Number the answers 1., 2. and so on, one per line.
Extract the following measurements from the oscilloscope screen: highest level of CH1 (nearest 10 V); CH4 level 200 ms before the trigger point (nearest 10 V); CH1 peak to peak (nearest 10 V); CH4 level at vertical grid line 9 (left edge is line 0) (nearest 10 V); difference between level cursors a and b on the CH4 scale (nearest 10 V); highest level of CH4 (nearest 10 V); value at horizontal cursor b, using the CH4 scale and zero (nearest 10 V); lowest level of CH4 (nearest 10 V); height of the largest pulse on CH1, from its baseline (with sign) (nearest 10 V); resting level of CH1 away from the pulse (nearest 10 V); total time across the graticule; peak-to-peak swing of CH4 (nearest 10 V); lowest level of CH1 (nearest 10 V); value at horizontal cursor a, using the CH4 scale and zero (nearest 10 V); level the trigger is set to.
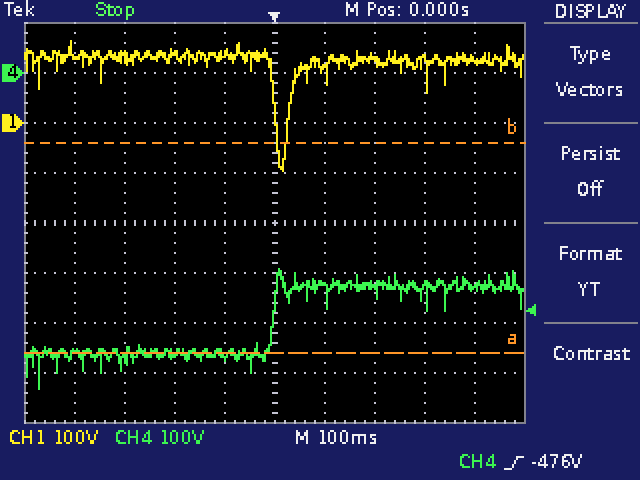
1. 160 V
2. -560 V
3. 260 V
4. -430 V
5. 420 V
6. -390 V
7. -140 V
8. -630 V
9. -230 V
10. 130 V
11. 1 s
12. 240 V
13. -100 V
14. -560 V
15. -476 V
